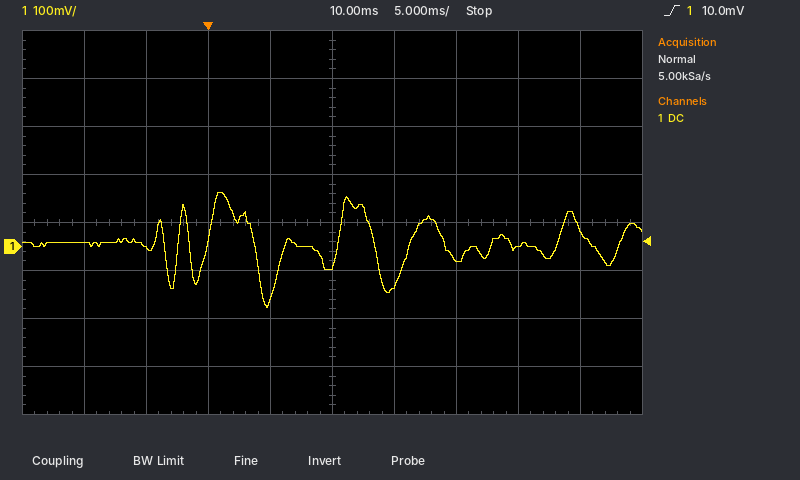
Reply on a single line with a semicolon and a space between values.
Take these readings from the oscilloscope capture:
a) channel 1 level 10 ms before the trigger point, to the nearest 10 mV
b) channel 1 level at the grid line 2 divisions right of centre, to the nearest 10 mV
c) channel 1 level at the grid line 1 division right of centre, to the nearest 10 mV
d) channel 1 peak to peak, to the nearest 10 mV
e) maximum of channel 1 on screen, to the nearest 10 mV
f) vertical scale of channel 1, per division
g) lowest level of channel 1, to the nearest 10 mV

10 mV; -30 mV; -80 mV; 240 mV; 110 mV; 100 mV; -130 mV
